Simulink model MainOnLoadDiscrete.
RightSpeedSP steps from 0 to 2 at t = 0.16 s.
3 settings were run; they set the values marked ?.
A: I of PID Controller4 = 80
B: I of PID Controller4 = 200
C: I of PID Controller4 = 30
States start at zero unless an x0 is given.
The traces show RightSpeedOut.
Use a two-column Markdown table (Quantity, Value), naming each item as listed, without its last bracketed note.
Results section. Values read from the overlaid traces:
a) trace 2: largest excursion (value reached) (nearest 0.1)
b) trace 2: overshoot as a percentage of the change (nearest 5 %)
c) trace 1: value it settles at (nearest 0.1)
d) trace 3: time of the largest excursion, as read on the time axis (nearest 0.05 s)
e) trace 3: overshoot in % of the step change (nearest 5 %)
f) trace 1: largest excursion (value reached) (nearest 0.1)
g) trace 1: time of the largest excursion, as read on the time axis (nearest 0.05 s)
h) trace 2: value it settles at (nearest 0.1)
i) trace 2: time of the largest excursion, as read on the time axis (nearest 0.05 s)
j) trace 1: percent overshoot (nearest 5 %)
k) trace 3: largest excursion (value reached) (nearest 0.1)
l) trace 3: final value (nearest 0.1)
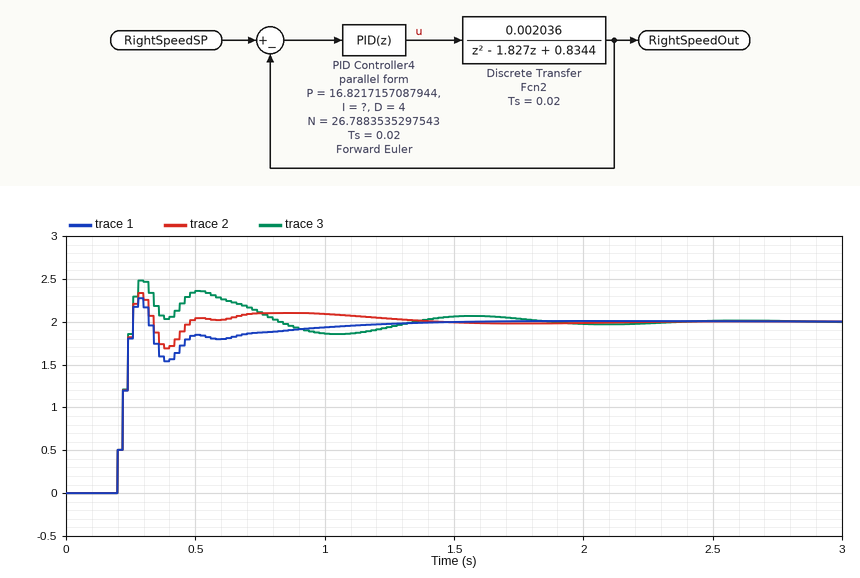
| Quantity | Value |
|---|---|
| trace 2: largest excursion (value reached) | 2.3 |
| trace 2: overshoot as a percentage of the change | 15 % |
| trace 1: value it settles at | 2.0 |
| trace 3: time of the largest excursion, as read on the time axis | 0.30 s |
| trace 3: overshoot in % of the step change | 25 % |
| trace 1: largest excursion (value reached) | 2.3 |
| trace 1: time of the largest excursion, as read on the time axis | 0.30 s |
| trace 2: value it settles at | 2.0 |
| trace 2: time of the largest excursion, as read on the time axis | 0.30 s |
| trace 1: percent overshoot | 15 % |
| trace 3: largest excursion (value reached) | 2.5 |
| trace 3: final value | 2.0 |
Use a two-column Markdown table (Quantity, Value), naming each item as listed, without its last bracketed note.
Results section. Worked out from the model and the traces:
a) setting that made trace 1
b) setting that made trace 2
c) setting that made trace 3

| Quantity | Value |
|---|---|
| setting that made trace 1 | C |
| setting that made trace 2 | A |
| setting that made trace 3 | B |
